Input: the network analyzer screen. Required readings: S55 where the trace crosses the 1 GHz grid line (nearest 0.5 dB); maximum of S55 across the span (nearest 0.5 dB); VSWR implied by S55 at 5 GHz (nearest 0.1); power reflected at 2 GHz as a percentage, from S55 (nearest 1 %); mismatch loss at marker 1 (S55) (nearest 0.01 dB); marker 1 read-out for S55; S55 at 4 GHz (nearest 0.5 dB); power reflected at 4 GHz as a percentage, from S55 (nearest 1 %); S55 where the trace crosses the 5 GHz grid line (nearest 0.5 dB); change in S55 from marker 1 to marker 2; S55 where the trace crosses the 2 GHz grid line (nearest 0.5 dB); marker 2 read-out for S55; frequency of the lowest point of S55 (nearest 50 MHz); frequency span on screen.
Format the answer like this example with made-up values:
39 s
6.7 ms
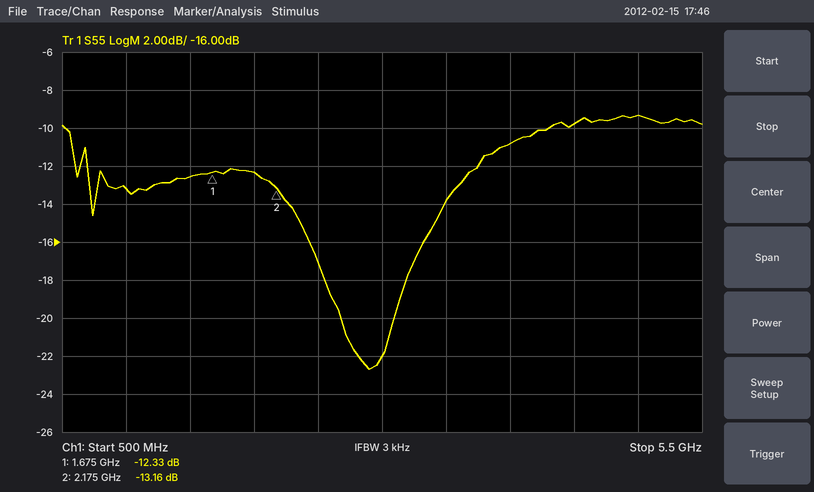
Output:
-13.0 dB
-9.5 dB
2.0
6 %
0.26 dB
-12.33 dB
-11.0 dB
8 %
-9.5 dB
-0.83 dB
-12.5 dB
-13.16 dB
2.90 GHz
5 GHz
